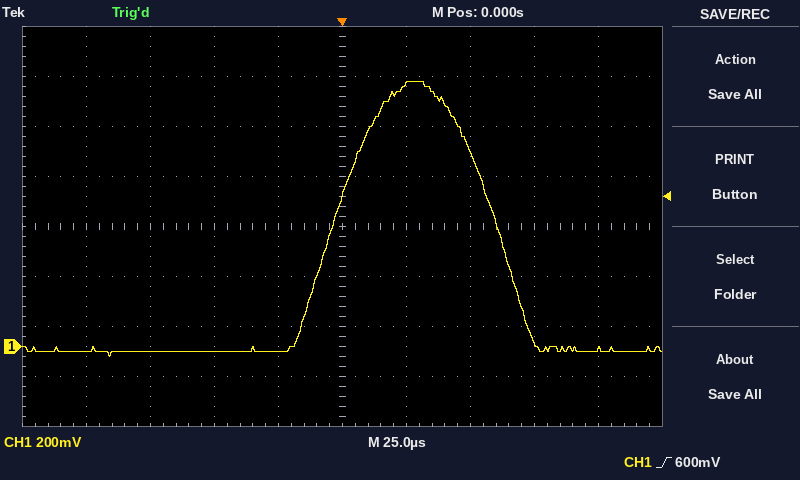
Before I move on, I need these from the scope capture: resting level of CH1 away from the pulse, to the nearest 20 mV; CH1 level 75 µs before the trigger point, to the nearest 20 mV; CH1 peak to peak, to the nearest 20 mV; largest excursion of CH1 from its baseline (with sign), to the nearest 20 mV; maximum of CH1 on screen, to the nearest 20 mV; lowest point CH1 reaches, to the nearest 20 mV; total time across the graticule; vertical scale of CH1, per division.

-20 mV
-20 mV
1.10 V
+1.08 V
1.06 V
-40 mV
250 µs
200 mV
